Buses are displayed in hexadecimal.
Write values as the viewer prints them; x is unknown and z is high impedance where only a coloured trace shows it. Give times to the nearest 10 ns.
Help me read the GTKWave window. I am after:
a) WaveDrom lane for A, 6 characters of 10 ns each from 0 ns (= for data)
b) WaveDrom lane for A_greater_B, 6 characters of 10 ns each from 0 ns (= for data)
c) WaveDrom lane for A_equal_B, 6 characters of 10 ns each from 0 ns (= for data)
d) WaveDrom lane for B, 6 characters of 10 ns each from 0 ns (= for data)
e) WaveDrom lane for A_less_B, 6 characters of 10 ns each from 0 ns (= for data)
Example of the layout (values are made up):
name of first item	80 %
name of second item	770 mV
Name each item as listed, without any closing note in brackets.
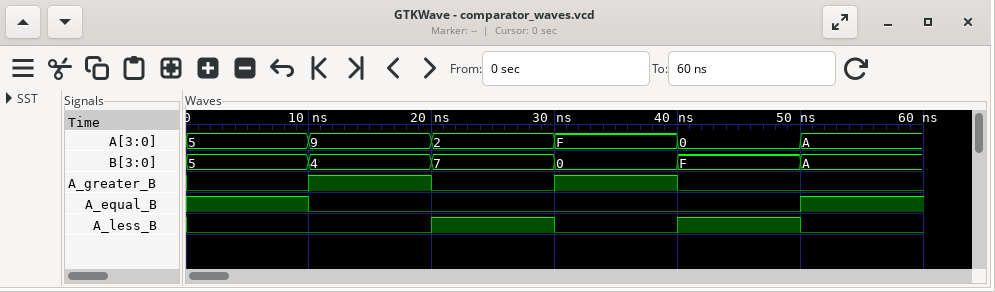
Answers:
WaveDrom lane for A, 6 characters of 10 ns each from 0 ns	{name: 'A', wave: '======', data: '5 9 2 F 0 A'}
WaveDrom lane for A_greater_B, 6 characters of 10 ns each from 0 ns	{name: 'A_greater_B', wave: '01010.'}
WaveDrom lane for A_equal_B, 6 characters of 10 ns each from 0 ns	{name: 'A_equal_B', wave: '10...1'}
WaveDrom lane for B, 6 characters of 10 ns each from 0 ns	{name: 'B', wave: '======', data: '5 4 7 0 F A'}
WaveDrom lane for A_less_B, 6 characters of 10 ns each from 0 ns	{name: 'A_less_B', wave: '0.1010'}
